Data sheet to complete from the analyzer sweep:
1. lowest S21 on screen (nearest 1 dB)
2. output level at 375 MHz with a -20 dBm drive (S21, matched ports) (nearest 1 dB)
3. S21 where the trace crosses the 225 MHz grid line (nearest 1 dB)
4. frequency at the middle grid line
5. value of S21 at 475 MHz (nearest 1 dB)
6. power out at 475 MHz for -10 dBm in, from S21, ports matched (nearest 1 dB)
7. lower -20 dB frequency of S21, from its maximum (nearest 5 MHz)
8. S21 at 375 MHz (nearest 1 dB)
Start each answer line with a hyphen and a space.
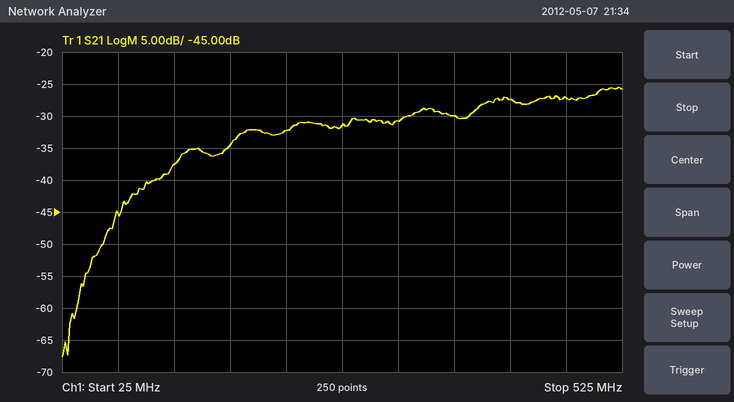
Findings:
- -68 dB
- -50 dBm
- -32 dB
- 275 MHz
- -27 dB
- -37 dBm
- 75 MHz
- -30 dB
